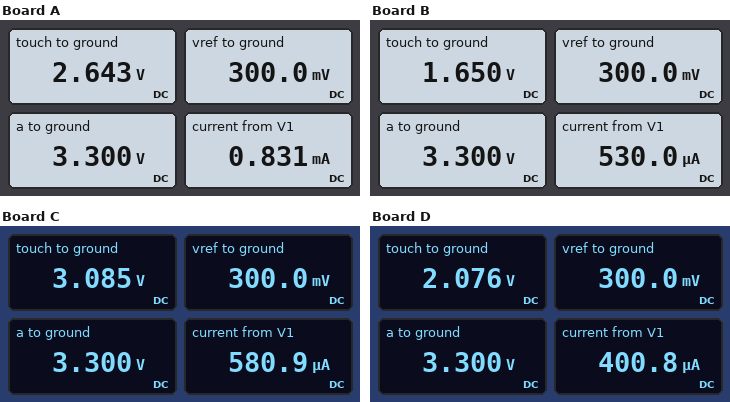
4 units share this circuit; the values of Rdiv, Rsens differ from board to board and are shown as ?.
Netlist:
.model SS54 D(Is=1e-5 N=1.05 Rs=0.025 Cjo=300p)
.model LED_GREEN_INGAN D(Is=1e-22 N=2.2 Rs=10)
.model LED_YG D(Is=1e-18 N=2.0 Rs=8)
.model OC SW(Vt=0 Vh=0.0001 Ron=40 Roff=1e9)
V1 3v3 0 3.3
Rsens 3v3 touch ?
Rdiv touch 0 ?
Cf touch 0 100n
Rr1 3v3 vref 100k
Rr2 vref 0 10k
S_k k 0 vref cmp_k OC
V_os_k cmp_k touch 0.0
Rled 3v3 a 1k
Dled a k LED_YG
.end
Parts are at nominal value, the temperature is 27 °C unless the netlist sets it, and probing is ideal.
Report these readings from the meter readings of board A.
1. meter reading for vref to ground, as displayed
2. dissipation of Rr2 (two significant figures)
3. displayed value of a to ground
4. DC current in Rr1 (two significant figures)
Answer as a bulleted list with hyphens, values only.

- 300.0 mV
- 9.0 µW
- 3.300 V
- 30 µA
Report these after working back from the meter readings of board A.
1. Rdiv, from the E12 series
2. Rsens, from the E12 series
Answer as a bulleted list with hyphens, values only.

- 3.3 kΩ
- 820 Ω
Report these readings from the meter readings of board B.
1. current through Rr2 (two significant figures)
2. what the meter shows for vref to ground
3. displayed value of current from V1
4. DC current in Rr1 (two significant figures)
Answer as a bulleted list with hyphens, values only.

- 30 µA
- 300.0 mV
- 530.0 µA
- 30 µA
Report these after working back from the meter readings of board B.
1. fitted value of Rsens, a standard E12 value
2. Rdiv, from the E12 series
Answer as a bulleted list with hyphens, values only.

- 3.3 kΩ
- 3.3 kΩ
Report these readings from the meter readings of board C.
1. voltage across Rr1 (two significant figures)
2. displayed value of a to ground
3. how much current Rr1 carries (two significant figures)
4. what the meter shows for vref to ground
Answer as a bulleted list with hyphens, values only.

- 3.0 V
- 3.300 V
- 30 µA
- 300.0 mV
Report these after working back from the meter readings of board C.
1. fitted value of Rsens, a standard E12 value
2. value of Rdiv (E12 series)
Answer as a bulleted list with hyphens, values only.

- 390 Ω
- 5.6 kΩ
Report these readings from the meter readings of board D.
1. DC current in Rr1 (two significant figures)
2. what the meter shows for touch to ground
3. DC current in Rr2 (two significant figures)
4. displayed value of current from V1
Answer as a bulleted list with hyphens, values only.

- 30 µA
- 2.076 V
- 30 µA
- 400.8 µA
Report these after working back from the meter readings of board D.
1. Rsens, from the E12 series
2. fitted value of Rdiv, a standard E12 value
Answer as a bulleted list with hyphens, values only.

- 3.3 kΩ
- 5.6 kΩ
